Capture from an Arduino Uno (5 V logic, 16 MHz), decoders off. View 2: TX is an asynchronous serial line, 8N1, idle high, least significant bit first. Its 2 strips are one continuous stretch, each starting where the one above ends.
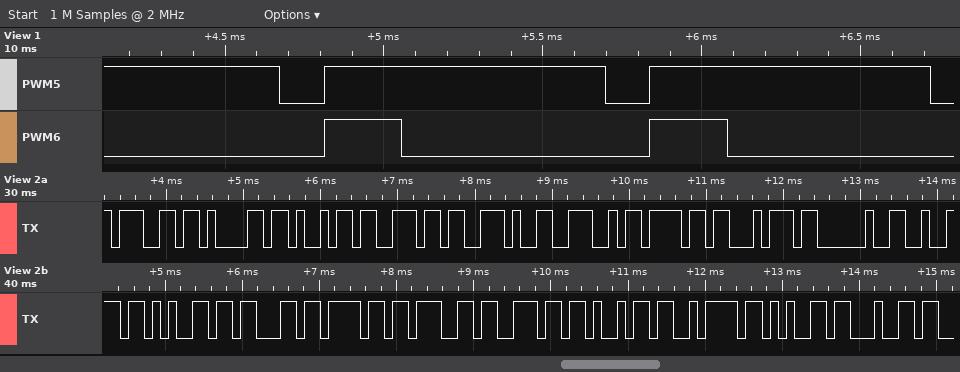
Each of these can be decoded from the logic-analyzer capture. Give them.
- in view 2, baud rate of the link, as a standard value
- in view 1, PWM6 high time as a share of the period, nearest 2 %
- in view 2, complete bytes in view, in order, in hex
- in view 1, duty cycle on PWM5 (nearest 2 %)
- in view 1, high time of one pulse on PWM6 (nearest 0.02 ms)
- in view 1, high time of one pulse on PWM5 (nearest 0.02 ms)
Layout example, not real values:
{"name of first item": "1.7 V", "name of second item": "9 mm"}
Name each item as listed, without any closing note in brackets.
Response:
{"in view 2, baud rate of the link, as a standard value": "9600 baud", "in view 1, PWM6 high time as a share of the period, nearest 2 %": "24 %", "in view 2, complete bytes in view, in order, in hex": "67 61 69 6E 2E 4E 6F 74 20 72 65 63 6F 67 6E 69 7A 65 64", "in view 1, duty cycle on PWM5": "86 %", "in view 1, high time of one pulse on PWM6": "0.24 ms", "in view 1, high time of one pulse on PWM5": "0.88 ms"}
